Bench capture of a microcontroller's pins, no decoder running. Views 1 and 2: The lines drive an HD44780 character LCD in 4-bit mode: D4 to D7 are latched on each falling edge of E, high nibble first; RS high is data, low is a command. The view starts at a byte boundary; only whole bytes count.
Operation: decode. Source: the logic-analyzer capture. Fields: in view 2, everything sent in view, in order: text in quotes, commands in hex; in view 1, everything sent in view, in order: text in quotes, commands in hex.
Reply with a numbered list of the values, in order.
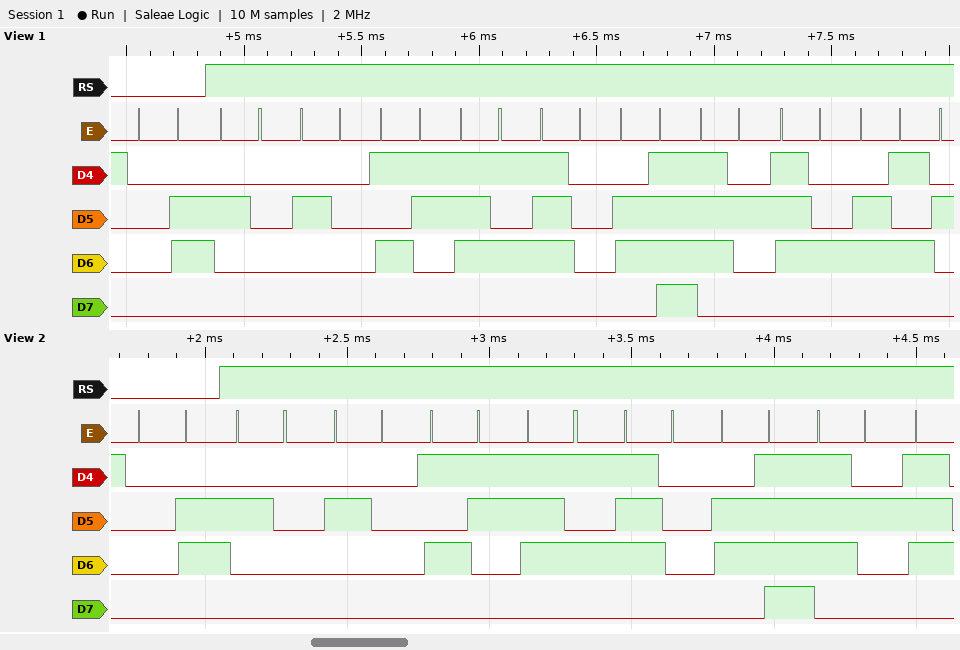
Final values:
1. 0x06 "  Supor"
2. 0x06 "  Suporte"
